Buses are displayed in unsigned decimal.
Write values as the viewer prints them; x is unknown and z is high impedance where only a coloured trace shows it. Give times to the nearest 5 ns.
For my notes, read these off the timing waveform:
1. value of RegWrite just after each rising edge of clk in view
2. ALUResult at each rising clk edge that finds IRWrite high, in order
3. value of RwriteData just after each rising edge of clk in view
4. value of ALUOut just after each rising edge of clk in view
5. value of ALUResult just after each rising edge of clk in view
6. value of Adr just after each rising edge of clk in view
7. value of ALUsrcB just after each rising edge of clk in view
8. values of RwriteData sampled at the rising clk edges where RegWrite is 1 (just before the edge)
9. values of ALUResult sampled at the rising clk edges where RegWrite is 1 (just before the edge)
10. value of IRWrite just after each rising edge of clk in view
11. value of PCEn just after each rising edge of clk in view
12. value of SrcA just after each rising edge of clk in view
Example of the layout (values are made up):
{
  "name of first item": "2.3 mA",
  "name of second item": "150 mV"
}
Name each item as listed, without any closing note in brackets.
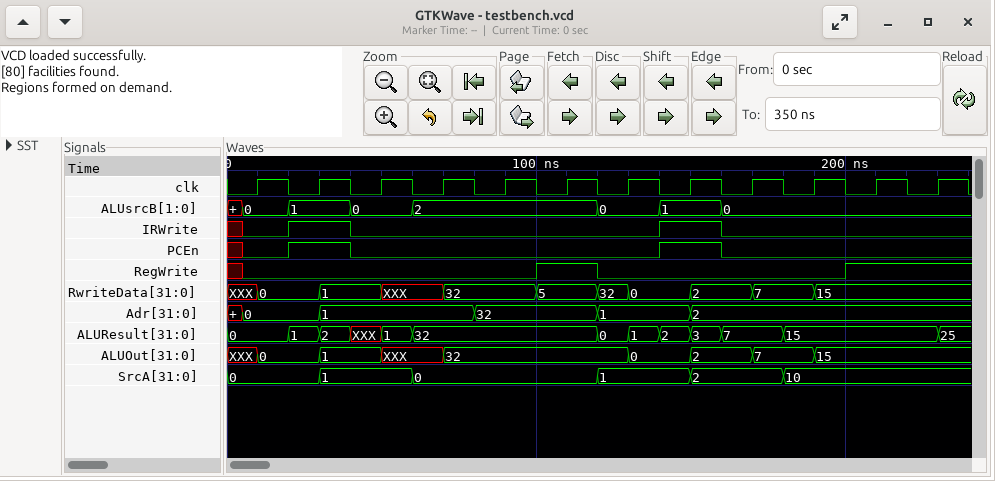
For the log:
{
  "value of RegWrite just after each rising edge of clk in view": "0 0 0 0 0 1 0 0 0 0 1 1",
  "ALUResult at each rising clk edge that finds IRWrite high, in order": "1, 2",
  "value of RwriteData just after each rising edge of clk in view": "0, 1, XXX, 32, 32, 5, 0, 2, 7, 15, 15, 15",
  "value of ALUOut just after each rising edge of clk in view": "0, 1, XXX, 32, 32, 32, 0, 2, 7, 15, 15, 15",
  "value of ALUResult just after each rising edge of clk in view": "0, 2, 1, 32, 32, 32, 1, 3, 7, 15, 15, 25",
  "value of Adr just after each rising edge of clk in view": "0, 1, 1, 1, 32, 32, 1, 2, 2, 2, 2, 2",
  "value of ALUsrcB just after each rising edge of clk in view": "0, 1, 0, 2, 2, 2, 0, 1, 0, 0, 0, 0",
  "values of RwriteData sampled at the rising clk edges where RegWrite is 1": "5, 15, 15",
  "values of ALUResult sampled at the rising clk edges where RegWrite is 1": "32, 15, 15",
  "value of IRWrite just after each rising edge of clk in view": "0 1 0 0 0 0 0 1 0 0 0 0",
  "value of PCEn just after each rising edge of clk in view": "0 1 0 0 0 0 0 1 0 0 0 0",
  "value of SrcA just after each rising edge of clk in view": "0, 1, 1, 0, 0, 0, 1, 2, 2, 10, 10, 10"
}
